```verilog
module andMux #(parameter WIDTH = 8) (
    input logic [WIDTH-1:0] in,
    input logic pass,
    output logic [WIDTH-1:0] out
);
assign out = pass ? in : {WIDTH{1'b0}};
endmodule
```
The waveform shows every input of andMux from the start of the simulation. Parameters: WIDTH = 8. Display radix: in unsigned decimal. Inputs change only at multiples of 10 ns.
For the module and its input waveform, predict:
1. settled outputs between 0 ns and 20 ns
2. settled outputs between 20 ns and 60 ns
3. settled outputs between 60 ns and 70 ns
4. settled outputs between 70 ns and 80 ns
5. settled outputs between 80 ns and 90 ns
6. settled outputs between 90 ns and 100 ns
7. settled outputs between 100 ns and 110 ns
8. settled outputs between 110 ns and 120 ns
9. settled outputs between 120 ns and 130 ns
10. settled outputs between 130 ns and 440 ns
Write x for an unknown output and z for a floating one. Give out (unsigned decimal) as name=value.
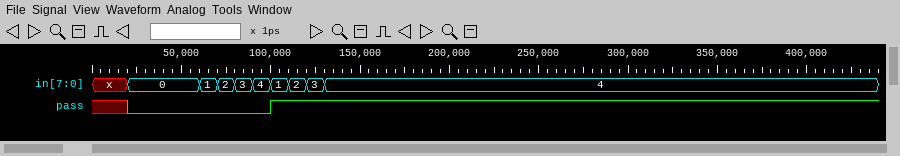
out=x
out=0
out=0
out=0
out=0
out=0
out=1
out=2
out=3
out=4
